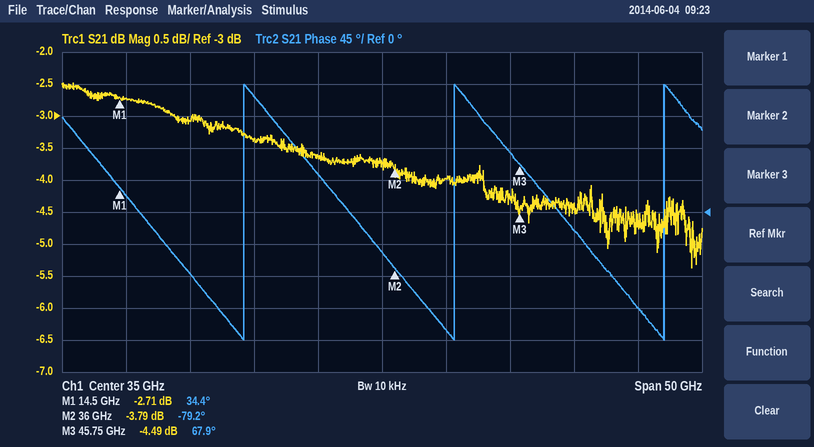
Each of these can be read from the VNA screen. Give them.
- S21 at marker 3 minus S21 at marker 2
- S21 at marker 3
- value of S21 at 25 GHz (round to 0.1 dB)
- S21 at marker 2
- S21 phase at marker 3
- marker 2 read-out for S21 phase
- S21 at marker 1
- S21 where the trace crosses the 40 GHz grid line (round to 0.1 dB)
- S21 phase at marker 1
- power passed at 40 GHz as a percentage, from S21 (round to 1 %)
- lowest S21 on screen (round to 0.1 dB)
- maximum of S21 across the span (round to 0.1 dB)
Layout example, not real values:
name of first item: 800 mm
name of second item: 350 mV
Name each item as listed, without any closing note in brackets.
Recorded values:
S21 at marker 3 minus S21 at marker 2: -0.70 dB
S21 at marker 3: -4.49 dB
value of S21 at 25 GHz: -3.4 dB
S21 at marker 2: -3.79 dB
S21 phase at marker 3: 67.9°
marker 2 read-out for S21 phase: -79.2°
S21 at marker 1: -2.71 dB
S21 where the trace crosses the 40 GHz grid line: -4.0 dB
S21 phase at marker 1: 34.4°
power passed at 40 GHz as a percentage, from S21: 40 %
lowest S21 on screen: -5.4 dB
maximum of S21 across the span: -2.5 dB
